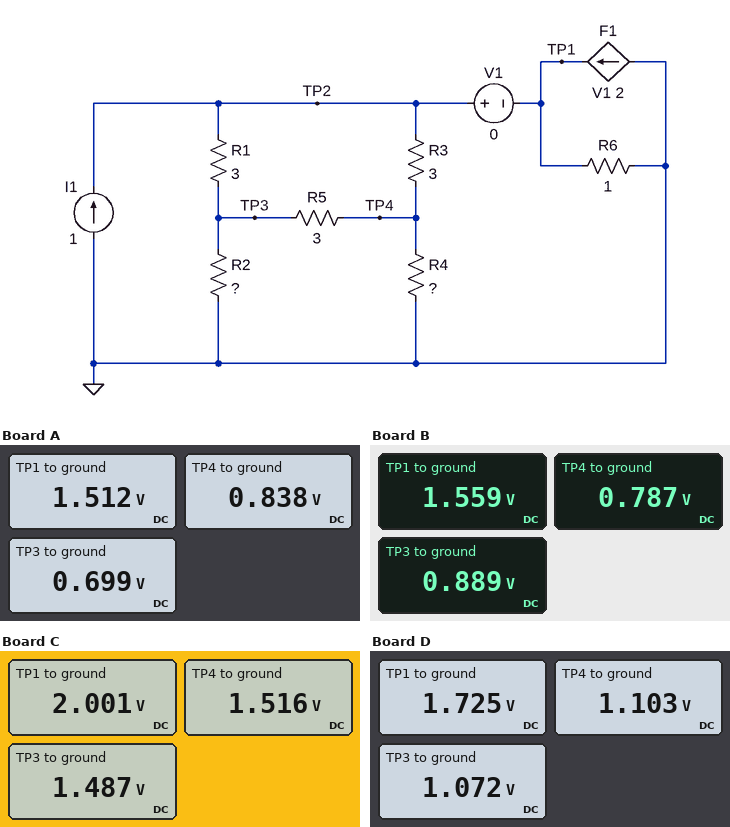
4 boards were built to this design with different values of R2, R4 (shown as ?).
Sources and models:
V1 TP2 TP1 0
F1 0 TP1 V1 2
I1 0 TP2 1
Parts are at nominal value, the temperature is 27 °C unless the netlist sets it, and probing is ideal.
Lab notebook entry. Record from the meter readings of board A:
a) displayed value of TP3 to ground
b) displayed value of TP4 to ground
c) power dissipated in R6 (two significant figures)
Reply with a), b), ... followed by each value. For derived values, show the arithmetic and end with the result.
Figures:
a) 0.699 V
b) 0.838 V
c) (1.512 V)^2 / 1 Ω = 2.3 W
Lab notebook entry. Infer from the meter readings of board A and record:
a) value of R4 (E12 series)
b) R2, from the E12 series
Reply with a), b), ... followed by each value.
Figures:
a) 4.7 Ω
b) 2.2 Ω
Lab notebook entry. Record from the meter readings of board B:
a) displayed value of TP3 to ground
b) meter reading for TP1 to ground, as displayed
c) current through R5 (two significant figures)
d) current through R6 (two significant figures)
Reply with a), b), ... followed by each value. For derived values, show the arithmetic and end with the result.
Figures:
a) 0.889 V
b) 1.559 V
c) (889 mV - 787 mV) / 3 Ω = 34 mA
d) (1.559 V) / 1 Ω = 1.6 A
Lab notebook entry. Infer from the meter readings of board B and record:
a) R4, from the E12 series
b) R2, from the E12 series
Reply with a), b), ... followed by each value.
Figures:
a) 2.7 Ω
b) 4.7 Ω
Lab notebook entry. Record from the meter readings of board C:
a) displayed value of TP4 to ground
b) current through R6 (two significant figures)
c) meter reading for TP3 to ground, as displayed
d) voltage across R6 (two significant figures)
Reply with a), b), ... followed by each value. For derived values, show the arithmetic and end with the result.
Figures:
a) 1.516 V
b) (2.001 V) / 1 Ω = 2.0 A
c) 1.487 V
d) 2.001 V = 2.0 V
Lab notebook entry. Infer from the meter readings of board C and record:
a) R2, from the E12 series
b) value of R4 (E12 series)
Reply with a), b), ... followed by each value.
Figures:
a) 8.2 Ω
b) 10 Ω
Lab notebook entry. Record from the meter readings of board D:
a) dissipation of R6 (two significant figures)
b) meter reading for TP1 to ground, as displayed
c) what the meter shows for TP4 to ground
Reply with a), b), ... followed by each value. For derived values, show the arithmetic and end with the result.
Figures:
a) (1.725 V)^2 / 1 Ω = 3.0 W
b) 1.725 V
c) 1.103 V
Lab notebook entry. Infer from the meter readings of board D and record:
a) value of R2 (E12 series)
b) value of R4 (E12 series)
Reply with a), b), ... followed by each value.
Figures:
a) 4.7 Ω
b) 5.6 Ω
